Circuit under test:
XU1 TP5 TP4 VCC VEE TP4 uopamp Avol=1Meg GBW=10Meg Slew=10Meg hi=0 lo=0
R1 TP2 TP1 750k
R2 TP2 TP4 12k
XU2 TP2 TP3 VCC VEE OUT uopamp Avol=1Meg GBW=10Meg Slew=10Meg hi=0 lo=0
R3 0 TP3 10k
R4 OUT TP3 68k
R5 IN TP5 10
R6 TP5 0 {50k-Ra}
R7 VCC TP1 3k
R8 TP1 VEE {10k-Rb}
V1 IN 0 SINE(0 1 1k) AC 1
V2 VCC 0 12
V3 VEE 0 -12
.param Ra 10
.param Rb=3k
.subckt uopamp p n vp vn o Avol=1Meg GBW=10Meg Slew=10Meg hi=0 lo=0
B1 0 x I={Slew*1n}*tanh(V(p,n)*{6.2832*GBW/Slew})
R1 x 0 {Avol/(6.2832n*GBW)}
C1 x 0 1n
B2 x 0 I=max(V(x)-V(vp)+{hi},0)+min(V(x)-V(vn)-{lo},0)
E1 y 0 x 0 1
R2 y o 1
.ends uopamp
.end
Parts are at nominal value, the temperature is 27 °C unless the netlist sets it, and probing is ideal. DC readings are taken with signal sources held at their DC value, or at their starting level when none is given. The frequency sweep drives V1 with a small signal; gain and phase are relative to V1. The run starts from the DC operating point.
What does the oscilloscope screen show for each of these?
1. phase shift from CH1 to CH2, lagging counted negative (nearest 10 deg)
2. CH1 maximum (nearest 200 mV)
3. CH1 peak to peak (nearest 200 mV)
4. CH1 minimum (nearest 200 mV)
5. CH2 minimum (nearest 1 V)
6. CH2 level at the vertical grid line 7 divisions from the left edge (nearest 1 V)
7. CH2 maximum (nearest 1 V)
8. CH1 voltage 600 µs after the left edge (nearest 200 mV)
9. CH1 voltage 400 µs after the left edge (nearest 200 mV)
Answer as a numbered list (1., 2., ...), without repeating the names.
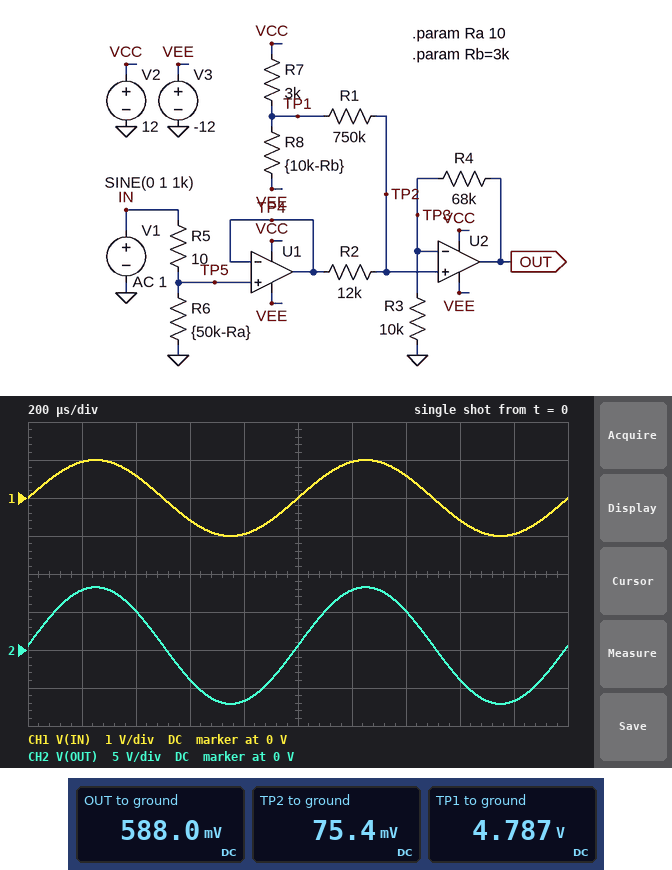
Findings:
1. 0 deg
2. 1.0 V
3. 2.0 V
4. -1.0 V
5. -7 V
6. 5 V
7. 8 V
8. -600 mV
9. 600 mV
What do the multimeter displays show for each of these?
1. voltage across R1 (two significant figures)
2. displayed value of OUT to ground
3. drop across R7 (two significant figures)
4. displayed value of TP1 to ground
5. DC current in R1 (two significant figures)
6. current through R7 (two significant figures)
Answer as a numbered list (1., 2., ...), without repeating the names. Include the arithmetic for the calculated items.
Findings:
1. 4.787 V - 75.4 mV = 4.7 V
2. 588.0 mV
3. 12 V - 4.787 V = 7.2 V
4. 4.787 V
5. (4.787 V - 75.4 mV) / 750 kΩ = 6.3 µA
6. (12 V - 4.787 V) / 3 kΩ = 2.4 mA
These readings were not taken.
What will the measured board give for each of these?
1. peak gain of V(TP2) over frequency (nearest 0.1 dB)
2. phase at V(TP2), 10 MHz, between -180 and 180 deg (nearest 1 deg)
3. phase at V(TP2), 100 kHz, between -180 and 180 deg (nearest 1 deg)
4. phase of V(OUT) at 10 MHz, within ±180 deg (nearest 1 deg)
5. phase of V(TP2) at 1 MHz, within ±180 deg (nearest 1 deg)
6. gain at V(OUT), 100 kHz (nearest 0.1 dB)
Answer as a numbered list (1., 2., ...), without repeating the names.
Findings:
1. -0.1 dB
2. -45 deg
3. -1 deg
4. -128 deg
5. -6 deg
6. 17.7 dB
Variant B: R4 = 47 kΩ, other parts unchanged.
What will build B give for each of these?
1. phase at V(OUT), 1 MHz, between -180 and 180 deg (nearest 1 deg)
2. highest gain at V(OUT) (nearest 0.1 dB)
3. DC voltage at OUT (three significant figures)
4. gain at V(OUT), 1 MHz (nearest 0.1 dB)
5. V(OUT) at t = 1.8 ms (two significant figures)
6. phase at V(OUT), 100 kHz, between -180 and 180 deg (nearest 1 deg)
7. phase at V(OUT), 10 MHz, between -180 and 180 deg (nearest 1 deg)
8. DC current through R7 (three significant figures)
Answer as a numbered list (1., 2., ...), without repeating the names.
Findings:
1. -35 deg
2. 15.0 dB
3. 430 mV
4. 13.7 dB
5. -4.9 V
6. -4 deg
7. -125 deg
8. 2.40 mA
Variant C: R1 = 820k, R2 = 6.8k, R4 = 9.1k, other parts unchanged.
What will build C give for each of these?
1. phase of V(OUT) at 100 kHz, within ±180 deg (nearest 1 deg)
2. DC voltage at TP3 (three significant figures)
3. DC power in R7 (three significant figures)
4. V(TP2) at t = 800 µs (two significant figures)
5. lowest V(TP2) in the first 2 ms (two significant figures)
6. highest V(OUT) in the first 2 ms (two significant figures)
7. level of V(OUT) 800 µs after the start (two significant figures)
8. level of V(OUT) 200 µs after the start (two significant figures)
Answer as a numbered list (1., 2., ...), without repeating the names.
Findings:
1. -2 deg
2. 39.4 mV
3. 17.3 mW
4. -900 mV
5. -950 mV
6. 2.0 V
7. -1.7 V
8. 1.9 V
